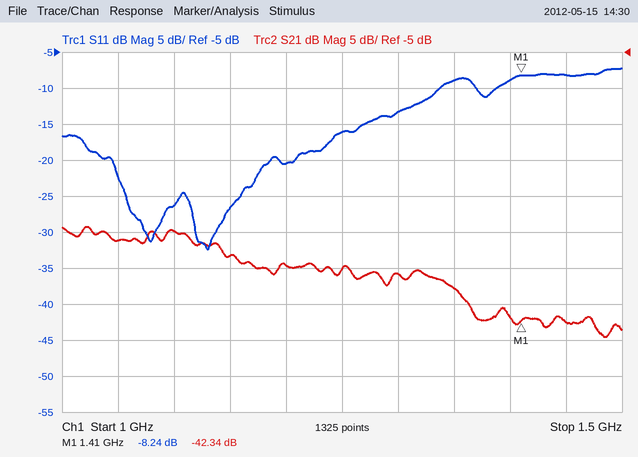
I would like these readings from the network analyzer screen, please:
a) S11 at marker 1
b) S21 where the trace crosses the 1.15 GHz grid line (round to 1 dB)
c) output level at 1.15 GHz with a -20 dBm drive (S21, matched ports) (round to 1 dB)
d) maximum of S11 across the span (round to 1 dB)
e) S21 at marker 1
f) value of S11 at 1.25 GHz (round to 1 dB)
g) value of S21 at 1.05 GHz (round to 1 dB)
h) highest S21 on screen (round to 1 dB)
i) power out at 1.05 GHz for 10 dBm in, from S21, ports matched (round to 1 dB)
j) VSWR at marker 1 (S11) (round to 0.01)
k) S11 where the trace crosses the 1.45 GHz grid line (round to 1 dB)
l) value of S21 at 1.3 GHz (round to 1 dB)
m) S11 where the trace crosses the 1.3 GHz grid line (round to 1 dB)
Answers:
-8.24 dB
-33 dB
-53 dBm
-7 dB
-42.34 dB
-16 dB
-31 dB
-29 dB
-21 dBm
2.26
-8 dB
-36 dB
-13 dB
